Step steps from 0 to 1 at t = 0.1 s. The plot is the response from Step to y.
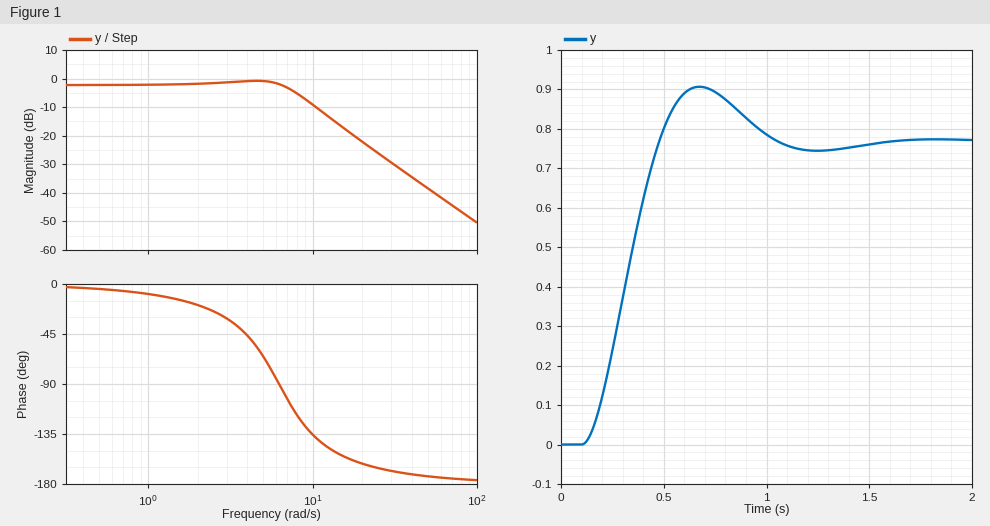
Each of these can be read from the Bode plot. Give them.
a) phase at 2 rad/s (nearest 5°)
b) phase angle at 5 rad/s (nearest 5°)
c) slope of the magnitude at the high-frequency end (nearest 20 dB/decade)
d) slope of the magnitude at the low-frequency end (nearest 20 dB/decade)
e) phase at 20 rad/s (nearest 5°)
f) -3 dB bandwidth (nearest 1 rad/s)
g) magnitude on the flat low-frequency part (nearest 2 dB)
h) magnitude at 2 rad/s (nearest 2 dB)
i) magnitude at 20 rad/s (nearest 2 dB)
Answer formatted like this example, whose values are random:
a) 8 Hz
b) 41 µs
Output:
a) -20°
b) -65°
c) -40 dB/decade
d) 0 dB/decade
e) -160°
f) 8 rad/s
g) -2 dB
h) -2 dB
i) -22 dB
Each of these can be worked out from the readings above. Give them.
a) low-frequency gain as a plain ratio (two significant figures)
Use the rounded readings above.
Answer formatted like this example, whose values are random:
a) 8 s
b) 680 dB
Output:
a) 0.79
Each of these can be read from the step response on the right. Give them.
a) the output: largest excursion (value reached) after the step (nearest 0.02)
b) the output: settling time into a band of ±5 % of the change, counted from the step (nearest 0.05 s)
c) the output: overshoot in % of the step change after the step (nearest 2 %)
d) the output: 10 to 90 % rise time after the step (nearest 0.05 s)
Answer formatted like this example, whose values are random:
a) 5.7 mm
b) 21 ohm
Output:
a) 0.90
b) 0.85 s
c) 18 %
d) 0.25 s
